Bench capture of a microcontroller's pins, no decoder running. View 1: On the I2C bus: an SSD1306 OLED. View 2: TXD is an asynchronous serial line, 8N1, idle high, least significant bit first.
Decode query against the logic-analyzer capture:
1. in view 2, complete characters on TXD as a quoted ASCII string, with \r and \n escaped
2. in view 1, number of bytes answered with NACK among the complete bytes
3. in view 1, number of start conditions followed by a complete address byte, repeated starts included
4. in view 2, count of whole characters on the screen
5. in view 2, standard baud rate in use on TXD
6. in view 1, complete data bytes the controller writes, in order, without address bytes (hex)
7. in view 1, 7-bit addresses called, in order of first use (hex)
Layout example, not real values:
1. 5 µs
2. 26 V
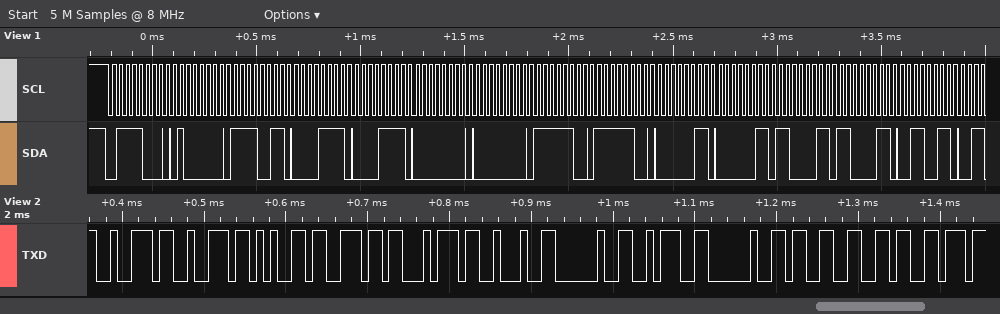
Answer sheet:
1. "rrent\" : 36"
2. 0
3. 1
4. 11
5. 115200 baud
6. 40 F3 0F 0F 00 00 FC FC 03 03 C3 C3 33
7. 0x3C
